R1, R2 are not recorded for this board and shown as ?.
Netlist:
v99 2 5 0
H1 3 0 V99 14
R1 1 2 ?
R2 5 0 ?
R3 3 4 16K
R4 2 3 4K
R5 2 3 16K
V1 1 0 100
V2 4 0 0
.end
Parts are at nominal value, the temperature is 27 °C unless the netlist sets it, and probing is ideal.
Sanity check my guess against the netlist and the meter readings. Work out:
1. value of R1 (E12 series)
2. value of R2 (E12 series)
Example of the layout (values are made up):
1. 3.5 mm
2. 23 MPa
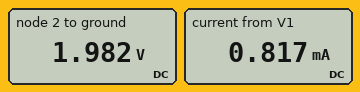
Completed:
1. 120 kΩ
2. 10 kΩ
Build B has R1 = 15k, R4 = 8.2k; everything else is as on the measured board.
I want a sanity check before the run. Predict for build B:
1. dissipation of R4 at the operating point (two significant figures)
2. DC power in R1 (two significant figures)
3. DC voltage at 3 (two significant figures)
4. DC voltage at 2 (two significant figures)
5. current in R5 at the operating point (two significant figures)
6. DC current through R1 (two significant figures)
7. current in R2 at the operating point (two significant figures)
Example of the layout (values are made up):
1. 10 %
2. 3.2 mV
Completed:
1. 44 mW
2. 440 mW
3. 27 mV
4. 19 V
5. 1.2 mA
6. 5.4 mA
7. 1.9 mA
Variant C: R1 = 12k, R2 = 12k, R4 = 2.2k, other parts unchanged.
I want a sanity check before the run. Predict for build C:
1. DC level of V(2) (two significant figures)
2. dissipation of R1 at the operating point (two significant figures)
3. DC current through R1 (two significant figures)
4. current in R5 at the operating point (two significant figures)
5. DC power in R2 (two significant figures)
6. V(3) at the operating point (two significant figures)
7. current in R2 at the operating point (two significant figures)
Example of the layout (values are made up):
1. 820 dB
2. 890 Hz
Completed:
1. 12 V
2. 640 mW
3. 7.3 mA
4. 760 µA
5. 12 mW
6. 14 mV
7. 1.0 mA
